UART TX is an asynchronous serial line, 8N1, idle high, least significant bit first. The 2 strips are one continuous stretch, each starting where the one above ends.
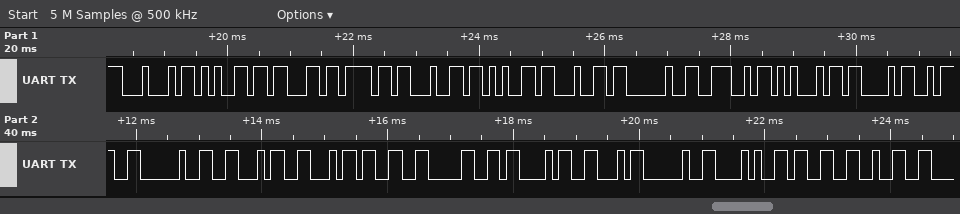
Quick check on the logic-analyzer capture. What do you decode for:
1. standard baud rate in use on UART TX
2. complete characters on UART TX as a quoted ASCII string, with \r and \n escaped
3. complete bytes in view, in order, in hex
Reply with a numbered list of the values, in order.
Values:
1. 9600 baud
2. "Decoded NEC: FF30CF (32"
3. 44 65 63 6F 64 65 64 20 4E 45 43 3A 20 46 46 33 30 43 46 20 28 33 32
